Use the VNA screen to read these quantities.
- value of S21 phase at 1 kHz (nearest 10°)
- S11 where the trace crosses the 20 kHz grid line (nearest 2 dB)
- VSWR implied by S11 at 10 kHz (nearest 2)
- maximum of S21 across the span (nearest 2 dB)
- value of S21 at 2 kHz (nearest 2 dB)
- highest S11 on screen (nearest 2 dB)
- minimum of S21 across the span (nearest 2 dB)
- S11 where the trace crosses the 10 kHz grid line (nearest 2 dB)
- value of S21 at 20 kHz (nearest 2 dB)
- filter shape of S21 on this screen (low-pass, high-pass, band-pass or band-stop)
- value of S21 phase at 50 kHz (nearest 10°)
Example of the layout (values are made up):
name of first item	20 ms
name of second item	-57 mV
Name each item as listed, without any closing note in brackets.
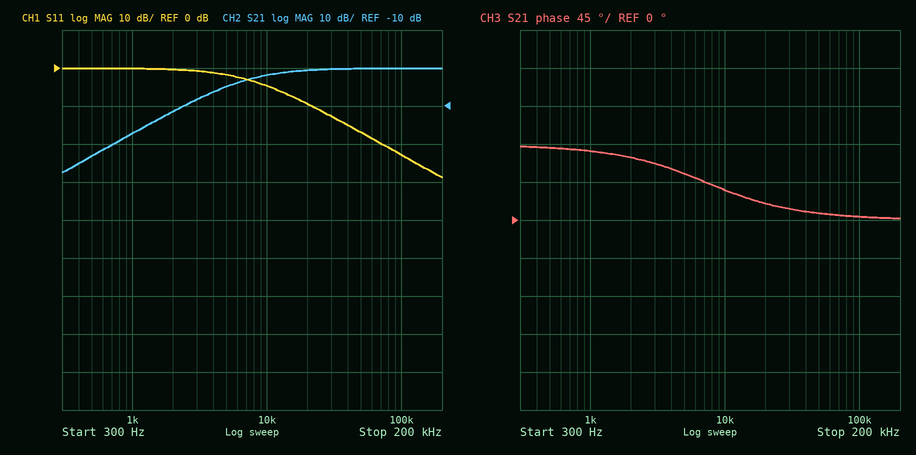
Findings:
value of S21 phase at 1 kHz	80°
S11 where the trace crosses the 20 kHz grid line	-10 dB
VSWR implied by S11 at 10 kHz	4
maximum of S21 across the span	0 dB
value of S21 at 2 kHz	-12 dB
highest S11 on screen	0 dB
minimum of S21 across the span	-28 dB
S11 where the trace crosses the 10 kHz grid line	-4 dB
value of S21 at 20 kHz	0 dB
filter shape of S21 on this screen	high-pass
value of S21 phase at 50 kHz	10°
